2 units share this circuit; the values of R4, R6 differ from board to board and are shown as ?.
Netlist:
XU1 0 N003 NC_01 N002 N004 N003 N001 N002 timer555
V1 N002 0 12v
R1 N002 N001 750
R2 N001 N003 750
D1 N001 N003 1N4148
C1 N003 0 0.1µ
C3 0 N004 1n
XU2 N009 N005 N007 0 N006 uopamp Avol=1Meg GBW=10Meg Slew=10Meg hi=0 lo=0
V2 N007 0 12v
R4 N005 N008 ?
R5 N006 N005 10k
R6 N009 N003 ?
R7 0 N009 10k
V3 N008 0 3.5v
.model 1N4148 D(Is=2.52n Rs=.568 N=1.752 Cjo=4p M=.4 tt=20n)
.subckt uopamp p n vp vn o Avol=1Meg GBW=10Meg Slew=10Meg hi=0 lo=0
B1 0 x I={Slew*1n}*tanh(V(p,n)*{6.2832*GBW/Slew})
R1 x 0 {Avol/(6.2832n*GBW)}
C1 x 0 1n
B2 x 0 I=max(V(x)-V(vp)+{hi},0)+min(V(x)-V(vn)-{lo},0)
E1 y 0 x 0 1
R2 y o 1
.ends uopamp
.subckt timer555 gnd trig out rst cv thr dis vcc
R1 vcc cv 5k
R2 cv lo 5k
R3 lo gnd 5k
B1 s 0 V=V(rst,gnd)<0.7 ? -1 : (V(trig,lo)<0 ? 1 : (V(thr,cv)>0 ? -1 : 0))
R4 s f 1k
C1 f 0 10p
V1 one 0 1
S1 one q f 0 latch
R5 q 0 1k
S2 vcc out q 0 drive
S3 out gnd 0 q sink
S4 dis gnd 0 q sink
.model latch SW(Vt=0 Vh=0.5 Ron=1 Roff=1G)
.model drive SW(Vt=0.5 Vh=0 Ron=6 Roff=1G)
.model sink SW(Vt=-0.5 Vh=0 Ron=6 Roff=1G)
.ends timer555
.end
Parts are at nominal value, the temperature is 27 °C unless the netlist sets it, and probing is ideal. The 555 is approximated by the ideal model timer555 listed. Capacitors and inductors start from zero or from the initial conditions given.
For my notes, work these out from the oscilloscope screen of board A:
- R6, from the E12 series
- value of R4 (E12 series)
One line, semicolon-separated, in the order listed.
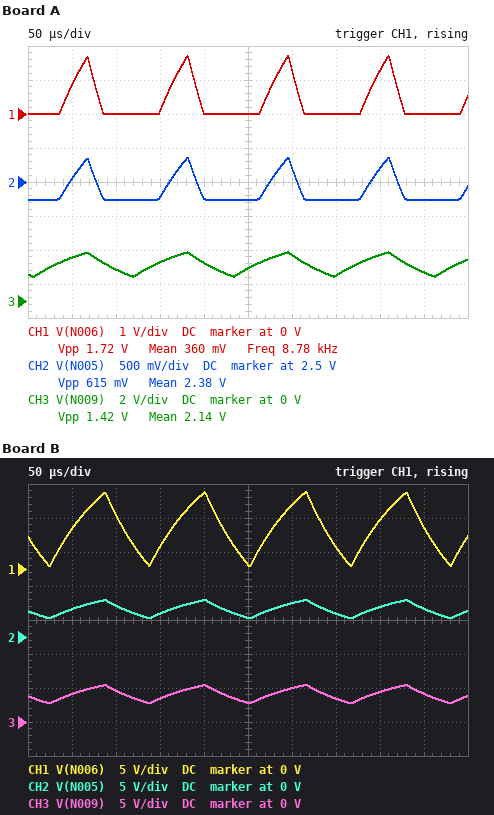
18 kΩ; 5.6 kΩ
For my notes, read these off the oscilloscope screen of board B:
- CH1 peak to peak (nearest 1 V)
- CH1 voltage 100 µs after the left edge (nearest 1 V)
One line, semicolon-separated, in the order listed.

11 V; 8 V
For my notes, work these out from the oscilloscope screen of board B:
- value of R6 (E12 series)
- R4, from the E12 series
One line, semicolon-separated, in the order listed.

4.7 kΩ; 3.3 kΩ
